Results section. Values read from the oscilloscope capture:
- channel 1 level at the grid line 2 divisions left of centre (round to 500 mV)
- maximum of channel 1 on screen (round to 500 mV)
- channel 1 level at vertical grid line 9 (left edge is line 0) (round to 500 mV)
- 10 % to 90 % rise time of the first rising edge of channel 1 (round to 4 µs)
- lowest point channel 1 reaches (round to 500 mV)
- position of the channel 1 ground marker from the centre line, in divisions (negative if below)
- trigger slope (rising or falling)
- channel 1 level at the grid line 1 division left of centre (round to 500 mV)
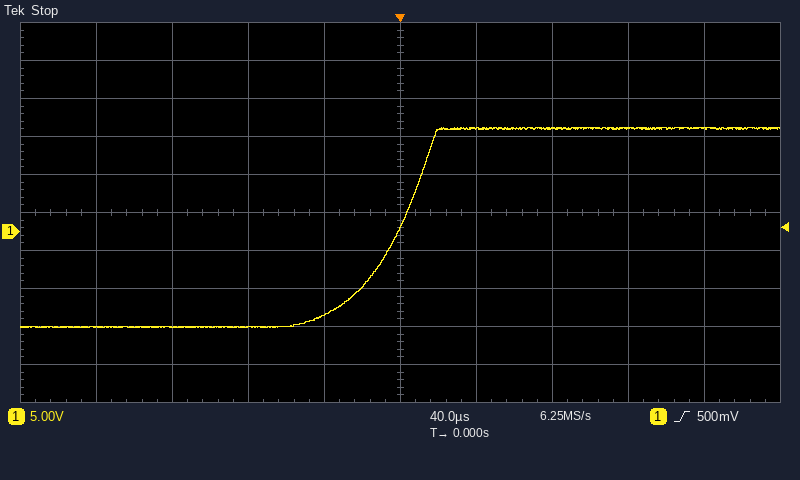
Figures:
-12.5 V
13.5 V
13.5 V
48 µs
-12.5 V
-0.5 div
rising
-11.0 V
